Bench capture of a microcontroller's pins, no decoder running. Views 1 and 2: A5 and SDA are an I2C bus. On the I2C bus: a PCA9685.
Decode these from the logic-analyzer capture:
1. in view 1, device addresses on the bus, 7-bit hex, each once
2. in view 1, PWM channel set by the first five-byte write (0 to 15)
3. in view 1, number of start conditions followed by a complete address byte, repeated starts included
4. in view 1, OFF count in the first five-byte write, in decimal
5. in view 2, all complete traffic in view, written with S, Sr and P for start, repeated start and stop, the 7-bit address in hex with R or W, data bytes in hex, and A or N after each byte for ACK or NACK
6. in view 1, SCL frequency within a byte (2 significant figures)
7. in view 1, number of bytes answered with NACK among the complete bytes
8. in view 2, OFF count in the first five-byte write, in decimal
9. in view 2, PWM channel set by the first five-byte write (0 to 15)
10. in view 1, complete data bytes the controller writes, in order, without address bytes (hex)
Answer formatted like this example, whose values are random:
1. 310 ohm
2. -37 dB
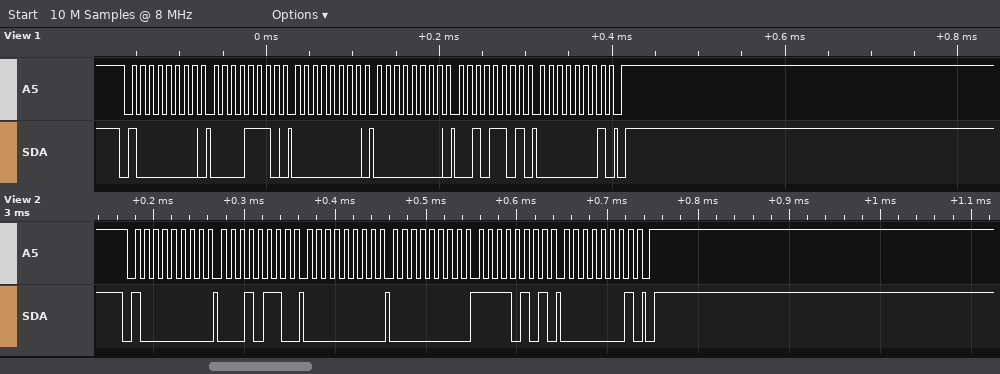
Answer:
1. 0x40
2. 2
3. 1
4. 301
5. S 40W A 16 A 00 A 00 A F5 A 01 A P
6. 100 kHz
7. 0
8. 501
9. 4
10. 0E 00 00 2D 01
